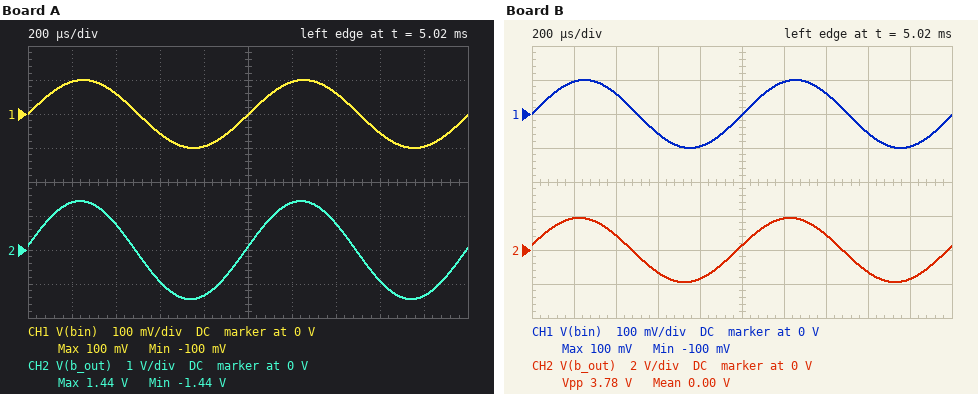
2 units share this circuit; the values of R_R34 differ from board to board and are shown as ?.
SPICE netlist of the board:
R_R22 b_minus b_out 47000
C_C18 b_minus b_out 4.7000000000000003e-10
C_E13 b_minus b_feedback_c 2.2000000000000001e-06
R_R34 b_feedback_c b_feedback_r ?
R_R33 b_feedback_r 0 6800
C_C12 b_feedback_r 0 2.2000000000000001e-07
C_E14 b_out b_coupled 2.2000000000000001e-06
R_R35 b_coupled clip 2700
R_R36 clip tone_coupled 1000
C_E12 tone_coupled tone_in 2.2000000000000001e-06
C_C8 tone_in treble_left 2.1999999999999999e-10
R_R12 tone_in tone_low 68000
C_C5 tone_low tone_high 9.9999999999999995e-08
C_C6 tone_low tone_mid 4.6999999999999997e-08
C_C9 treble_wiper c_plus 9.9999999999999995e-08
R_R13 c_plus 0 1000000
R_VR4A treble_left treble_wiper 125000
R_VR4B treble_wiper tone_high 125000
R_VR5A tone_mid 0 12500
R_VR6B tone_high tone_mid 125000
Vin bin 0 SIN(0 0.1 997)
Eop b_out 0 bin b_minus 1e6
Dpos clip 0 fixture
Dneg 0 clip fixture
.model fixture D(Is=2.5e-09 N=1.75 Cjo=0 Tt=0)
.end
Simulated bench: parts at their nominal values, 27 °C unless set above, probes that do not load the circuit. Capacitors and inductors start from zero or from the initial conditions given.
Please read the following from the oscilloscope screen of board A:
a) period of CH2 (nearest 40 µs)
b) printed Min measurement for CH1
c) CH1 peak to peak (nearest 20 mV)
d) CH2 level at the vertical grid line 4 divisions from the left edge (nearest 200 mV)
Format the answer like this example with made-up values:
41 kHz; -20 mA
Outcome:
1.00 ms; -100 mV; 200 mV; -1.4 V
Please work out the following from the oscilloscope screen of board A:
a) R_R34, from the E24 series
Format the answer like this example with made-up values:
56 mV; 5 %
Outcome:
3.3 kΩ
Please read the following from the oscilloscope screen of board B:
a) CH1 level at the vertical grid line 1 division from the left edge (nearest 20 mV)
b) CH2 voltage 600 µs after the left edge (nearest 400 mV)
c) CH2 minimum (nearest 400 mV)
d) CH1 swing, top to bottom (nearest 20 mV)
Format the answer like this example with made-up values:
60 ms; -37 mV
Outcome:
100 mV; -1.2 V; -2.0 V; 200 mV
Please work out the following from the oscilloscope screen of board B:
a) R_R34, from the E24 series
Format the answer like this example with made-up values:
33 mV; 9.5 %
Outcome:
2.4 kΩ
